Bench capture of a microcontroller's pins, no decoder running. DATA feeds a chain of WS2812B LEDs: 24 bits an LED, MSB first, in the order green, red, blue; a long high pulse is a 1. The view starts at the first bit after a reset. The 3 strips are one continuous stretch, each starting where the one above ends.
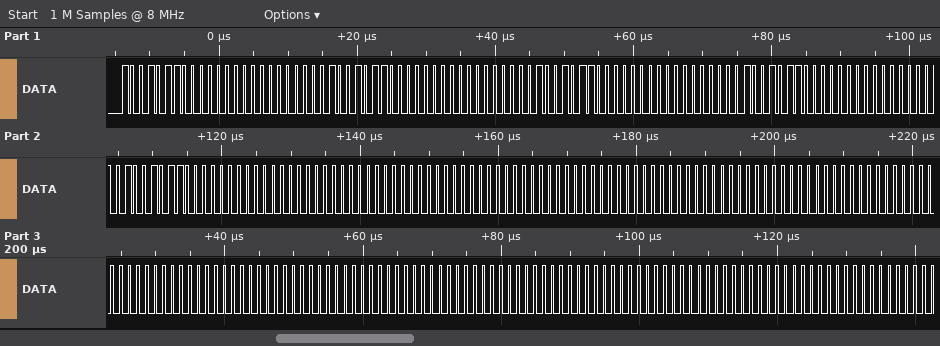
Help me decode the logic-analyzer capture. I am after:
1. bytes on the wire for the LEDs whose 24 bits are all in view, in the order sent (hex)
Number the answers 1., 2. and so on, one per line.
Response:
1. 96 00 00 96 00 00 96 00 00 96 00 00 96 00 00 00 00 00 00 00 00 00 00 00 00 00 00 00 00 00 00 00 00
